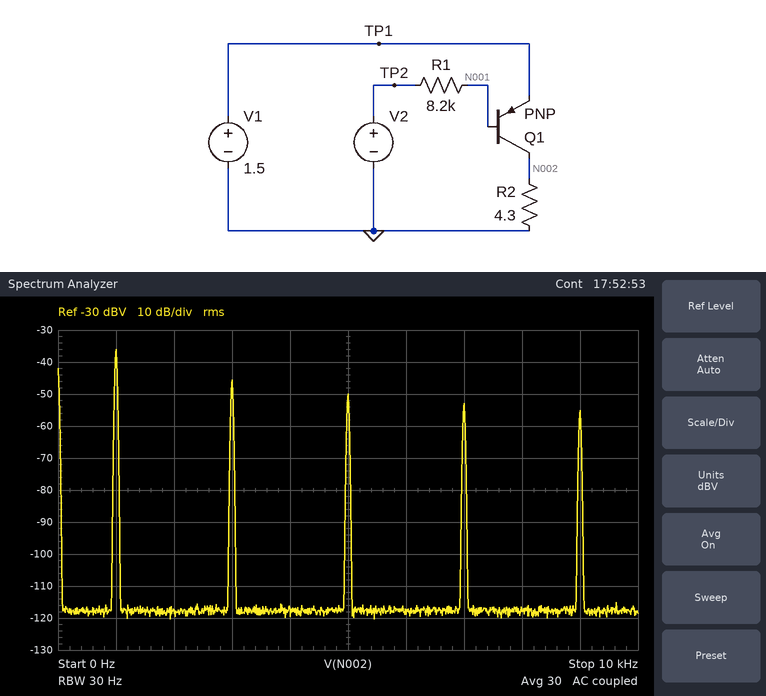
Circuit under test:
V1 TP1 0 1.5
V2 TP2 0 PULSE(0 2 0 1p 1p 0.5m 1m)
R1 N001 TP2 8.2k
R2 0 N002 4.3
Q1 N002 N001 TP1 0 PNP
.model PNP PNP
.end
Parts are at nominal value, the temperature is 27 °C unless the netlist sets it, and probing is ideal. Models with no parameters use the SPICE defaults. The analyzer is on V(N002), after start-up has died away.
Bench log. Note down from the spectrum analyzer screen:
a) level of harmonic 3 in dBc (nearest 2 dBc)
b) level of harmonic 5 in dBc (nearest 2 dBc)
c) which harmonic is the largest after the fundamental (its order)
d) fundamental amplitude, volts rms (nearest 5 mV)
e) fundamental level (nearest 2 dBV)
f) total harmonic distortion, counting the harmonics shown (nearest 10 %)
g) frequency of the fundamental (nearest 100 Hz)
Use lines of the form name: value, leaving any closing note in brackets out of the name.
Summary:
level of harmonic 3 in dBc: -10 dBc
level of harmonic 5 in dBc: -14 dBc
which harmonic is the largest after the fundamental: 3
fundamental amplitude, volts rms: 15 mV
fundamental level: -36 dBV
total harmonic distortion, counting the harmonics shown: 40 %
frequency of the fundamental: 1.0 kHz
